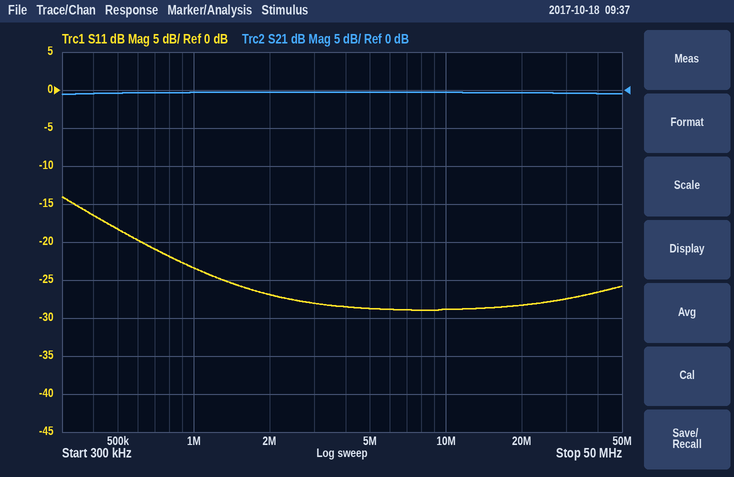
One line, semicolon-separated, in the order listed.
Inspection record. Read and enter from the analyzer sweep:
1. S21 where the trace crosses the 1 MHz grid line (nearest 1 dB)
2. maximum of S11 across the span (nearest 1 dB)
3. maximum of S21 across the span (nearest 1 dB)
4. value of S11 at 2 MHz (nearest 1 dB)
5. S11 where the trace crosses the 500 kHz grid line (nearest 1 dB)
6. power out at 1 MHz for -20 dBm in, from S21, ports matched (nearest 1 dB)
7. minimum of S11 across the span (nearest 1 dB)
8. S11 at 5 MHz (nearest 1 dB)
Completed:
0 dB; -14 dB; 0 dB; -27 dB; -18 dB; -20 dBm; -29 dB; -29 dB
